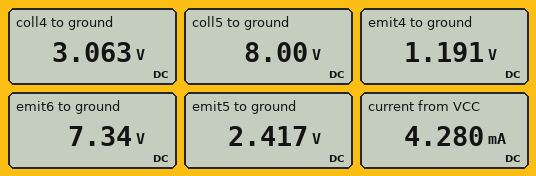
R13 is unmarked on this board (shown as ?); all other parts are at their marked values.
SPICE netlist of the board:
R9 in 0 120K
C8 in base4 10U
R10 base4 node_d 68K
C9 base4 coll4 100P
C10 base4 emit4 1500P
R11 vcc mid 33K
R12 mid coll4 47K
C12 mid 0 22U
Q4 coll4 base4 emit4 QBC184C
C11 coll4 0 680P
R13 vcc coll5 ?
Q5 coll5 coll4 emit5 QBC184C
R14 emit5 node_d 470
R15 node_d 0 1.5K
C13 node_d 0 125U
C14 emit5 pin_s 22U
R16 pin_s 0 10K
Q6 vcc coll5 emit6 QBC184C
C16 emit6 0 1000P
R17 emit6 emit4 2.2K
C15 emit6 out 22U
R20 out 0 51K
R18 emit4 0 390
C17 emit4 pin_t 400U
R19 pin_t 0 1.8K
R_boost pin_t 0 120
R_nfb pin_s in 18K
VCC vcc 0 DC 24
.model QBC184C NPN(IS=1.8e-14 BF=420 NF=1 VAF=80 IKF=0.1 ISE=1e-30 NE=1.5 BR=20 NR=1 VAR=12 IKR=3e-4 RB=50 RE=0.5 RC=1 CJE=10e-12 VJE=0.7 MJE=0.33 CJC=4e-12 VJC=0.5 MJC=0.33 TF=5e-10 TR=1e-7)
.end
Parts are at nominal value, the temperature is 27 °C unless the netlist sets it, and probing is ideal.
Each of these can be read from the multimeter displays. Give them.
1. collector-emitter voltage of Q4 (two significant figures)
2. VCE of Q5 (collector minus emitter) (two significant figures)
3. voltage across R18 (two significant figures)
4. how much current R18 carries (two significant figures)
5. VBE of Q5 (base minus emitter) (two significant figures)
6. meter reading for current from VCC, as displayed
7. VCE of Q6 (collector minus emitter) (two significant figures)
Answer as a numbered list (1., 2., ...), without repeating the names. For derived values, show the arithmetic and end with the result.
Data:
1. 3.063 V - 1.191 V = 1.9 V
2. 8 V - 2.417 V = 5.6 V
3. 1.191 V = 1.2 V
4. (1.191 V) / 390 Ω = 3.1 mA
5. 3.063 V - 2.417 V = 650 mV
6. 4.280 mA
7. 24 V - 7.34 V = 17 V
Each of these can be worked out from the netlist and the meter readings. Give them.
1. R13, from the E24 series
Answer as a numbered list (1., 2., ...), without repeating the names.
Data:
1. 13 kΩ
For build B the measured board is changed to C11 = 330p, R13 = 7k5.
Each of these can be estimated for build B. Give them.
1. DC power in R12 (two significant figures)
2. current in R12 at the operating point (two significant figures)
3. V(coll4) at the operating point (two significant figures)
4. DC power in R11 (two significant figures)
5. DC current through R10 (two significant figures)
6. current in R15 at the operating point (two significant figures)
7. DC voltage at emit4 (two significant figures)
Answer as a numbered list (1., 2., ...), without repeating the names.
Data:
1. 3.0 mW
2. 250 µA
3. 3.8 V
4. 2.1 mW
5. 610 nA
6. 1.6 mA
7. 1.8 V
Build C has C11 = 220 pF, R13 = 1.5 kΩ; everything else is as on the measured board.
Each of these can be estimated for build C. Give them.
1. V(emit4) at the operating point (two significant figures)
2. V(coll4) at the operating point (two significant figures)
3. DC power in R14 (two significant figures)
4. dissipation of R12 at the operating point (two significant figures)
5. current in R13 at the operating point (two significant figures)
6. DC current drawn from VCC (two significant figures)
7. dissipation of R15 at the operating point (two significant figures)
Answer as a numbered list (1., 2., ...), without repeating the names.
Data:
1. 3.0 V
2. 5.5 V
3. 2.8 mW
4. 2.5 mW
5. 2.5 mA
6. 10 mA
7. 9.0 mW
